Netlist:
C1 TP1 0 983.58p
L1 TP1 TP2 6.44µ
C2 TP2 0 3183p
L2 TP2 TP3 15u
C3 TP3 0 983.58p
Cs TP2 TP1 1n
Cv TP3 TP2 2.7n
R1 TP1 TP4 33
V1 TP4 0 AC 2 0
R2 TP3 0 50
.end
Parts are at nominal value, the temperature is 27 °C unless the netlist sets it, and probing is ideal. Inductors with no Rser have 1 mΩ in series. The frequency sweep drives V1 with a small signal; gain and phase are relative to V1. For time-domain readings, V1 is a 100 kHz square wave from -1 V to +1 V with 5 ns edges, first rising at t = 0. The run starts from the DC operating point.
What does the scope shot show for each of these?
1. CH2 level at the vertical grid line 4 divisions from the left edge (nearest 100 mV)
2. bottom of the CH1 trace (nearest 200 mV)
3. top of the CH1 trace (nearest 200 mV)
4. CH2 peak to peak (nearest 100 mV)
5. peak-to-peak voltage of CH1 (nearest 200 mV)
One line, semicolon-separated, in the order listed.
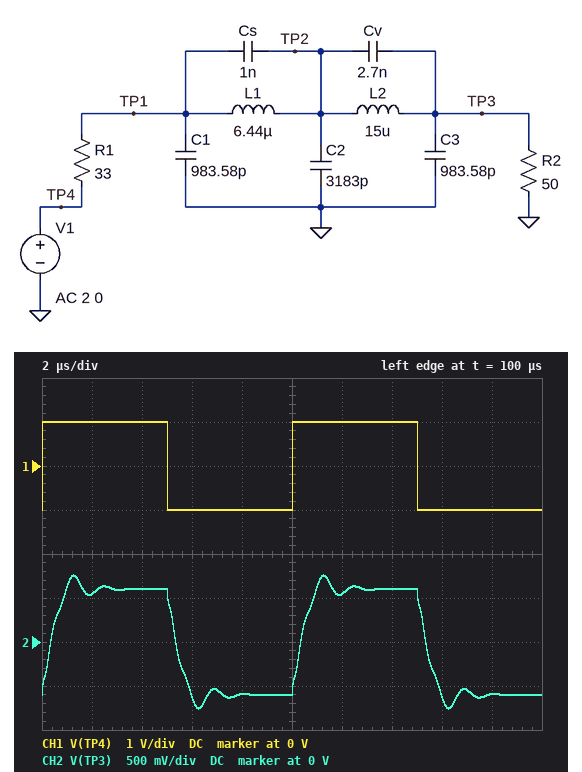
-600 mV; -1.0 V; 1.0 V; 1.5 V; 2.0 V
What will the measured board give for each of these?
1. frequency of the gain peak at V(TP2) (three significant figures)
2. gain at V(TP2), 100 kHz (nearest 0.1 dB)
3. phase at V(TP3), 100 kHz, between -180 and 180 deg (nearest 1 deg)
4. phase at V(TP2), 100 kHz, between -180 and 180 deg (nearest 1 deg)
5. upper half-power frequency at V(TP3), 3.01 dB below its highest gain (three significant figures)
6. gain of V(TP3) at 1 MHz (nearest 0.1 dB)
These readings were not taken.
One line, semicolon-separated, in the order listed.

833 kHz; -4.3 dB; -13 deg; -2 deg; 548 kHz; -10.6 dB
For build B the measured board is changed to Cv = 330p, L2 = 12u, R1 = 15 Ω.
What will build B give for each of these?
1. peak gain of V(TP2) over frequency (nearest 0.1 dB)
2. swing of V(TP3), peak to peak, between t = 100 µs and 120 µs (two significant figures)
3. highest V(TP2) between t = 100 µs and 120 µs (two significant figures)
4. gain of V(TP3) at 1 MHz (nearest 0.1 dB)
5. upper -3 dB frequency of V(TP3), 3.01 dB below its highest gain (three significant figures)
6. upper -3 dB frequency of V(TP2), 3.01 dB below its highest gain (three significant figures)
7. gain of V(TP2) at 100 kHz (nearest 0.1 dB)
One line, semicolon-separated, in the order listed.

6.0 dB; 1.8 V; 1.3 V; -2.4 dB; 1.25 MHz; 1.27 MHz; -2.3 dB
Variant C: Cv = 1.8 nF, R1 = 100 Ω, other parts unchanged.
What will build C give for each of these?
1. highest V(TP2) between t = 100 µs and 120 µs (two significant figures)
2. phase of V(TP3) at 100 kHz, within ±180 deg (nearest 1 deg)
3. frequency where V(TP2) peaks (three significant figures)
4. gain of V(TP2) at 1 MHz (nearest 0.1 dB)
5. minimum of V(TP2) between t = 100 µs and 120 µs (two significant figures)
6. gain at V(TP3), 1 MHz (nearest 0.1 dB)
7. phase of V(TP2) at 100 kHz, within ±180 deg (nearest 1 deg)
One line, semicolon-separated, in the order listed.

720 mV; -11 deg; 693 kHz; -6.0 dB; -720 mV; -35.6 dB; -1 deg
